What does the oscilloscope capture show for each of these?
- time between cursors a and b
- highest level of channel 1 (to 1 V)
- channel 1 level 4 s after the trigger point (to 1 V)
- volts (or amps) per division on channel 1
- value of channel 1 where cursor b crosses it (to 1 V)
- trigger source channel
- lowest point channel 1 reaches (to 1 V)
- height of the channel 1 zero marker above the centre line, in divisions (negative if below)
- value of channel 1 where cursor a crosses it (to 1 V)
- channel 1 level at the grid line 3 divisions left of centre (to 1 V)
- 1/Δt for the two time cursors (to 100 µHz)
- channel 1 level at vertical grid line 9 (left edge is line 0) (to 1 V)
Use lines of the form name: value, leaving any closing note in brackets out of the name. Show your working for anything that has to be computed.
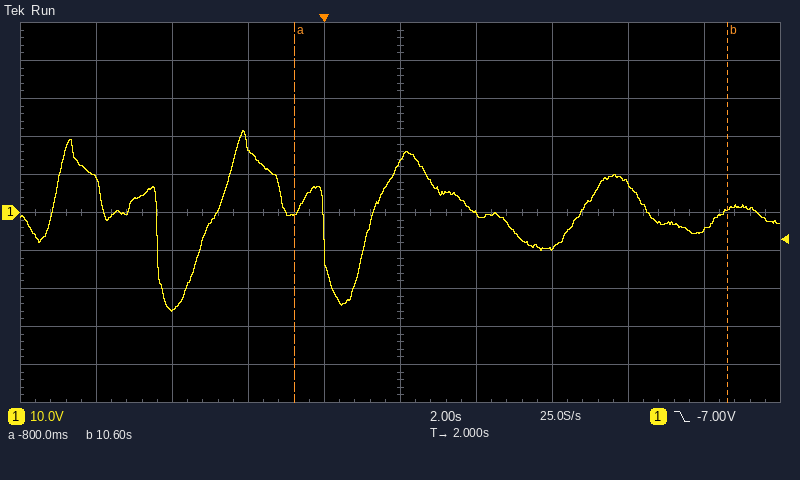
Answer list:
time between cursors a and b: 10.6 s − (-800 ms) = 11.4 s
highest level of channel 1: 22 V
channel 1 level 4 s after the trigger point: 0 V
volts (or amps) per division on channel 1: 10 V
value of channel 1 where cursor b crosses it: 1 V
trigger source channel: channel 1
lowest point channel 1 reaches: -26 V
height of the channel 1 zero marker above the centre line, in divisions: 0.0 div
value of channel 1 where cursor a crosses it: 0 V
channel 1 level at the grid line 3 divisions left of centre: -25 V
1/Δt for the two time cursors: 1 / 11.4 s ≈ 87.7 mHz
channel 1 level at vertical grid line 9 (left edge is line 0): -5 V
